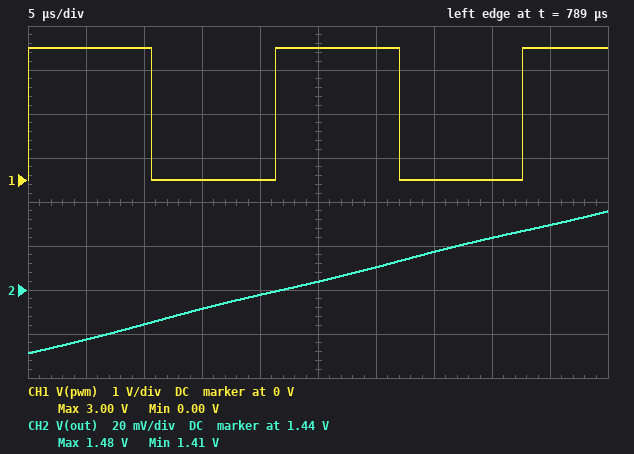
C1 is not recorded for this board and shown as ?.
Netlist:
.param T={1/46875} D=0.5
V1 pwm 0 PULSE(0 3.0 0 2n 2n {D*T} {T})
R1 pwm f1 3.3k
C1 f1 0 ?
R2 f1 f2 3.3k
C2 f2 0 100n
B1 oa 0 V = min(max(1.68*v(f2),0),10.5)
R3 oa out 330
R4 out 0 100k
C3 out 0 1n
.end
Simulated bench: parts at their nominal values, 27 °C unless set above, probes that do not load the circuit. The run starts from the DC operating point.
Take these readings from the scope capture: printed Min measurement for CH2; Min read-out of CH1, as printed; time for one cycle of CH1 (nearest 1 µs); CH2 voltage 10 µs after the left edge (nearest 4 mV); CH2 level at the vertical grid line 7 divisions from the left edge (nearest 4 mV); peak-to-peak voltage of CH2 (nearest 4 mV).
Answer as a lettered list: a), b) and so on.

a) 1.41 V
b) 0.00 V
c) 21 µs
d) 1.424 V
e) 1.456 V
f) 64 mV
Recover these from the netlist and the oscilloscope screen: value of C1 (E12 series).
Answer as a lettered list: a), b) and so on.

a) 82 nF
